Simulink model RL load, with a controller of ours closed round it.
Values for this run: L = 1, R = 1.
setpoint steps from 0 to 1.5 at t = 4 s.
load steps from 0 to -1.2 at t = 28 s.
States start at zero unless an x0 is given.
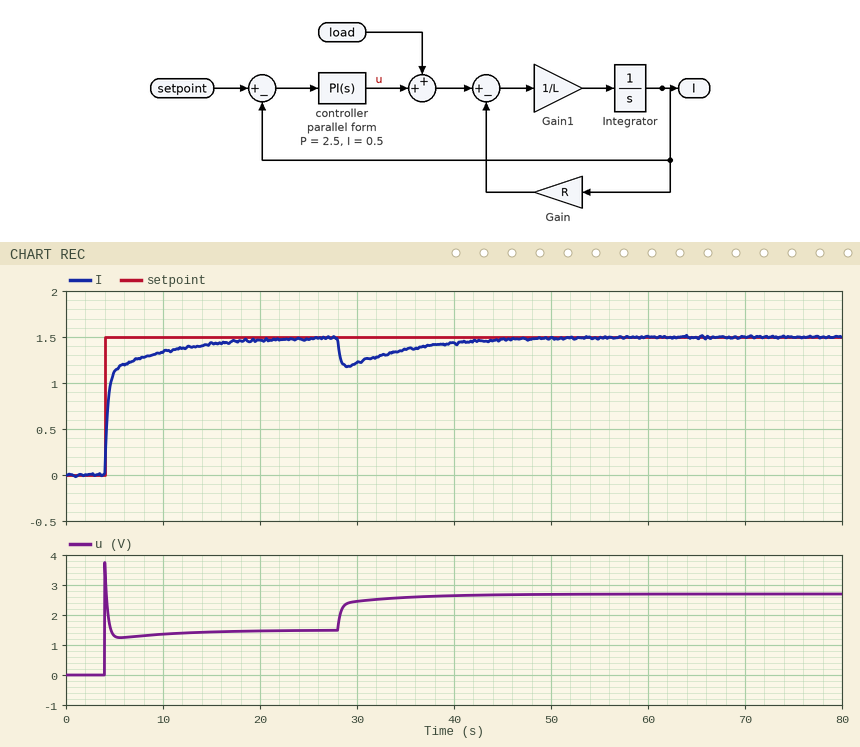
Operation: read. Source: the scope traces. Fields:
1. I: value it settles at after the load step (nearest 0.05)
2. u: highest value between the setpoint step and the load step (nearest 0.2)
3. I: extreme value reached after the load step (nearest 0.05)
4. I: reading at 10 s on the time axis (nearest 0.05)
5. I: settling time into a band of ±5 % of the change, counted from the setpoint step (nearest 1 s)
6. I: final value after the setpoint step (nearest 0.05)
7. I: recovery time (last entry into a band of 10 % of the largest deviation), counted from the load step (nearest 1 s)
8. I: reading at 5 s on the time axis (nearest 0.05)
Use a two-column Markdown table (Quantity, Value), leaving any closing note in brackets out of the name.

| Quantity | Value |
|---|---|
| I: value it settles at after the load step | 1.50 |
| u: highest value between the setpoint step and the load step | 3.8 |
| I: extreme value reached after the load step | 1.20 |
| I: reading at 10 s on the time axis | 1.35 |
| I: settling time into a band of ±5 % of the change, counted from the setpoint step | 11 s |
| I: final value after the setpoint step | 1.50 |
| I: recovery time (last entry into a band of 10 % of the largest deviation), counted from the load step | 17 s |
| I: reading at 5 s on the time axis | 1.10 |
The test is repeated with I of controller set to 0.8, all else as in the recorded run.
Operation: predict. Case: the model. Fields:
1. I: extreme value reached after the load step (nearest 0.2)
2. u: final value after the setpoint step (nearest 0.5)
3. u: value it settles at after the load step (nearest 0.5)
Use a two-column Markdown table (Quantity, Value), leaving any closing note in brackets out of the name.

| Quantity | Value |
|---|---|
| I: extreme value reached after the load step | 1.2 |
| u: final value after the setpoint step | 1.5 |
| u: value it settles at after the load step | 2.5 |
